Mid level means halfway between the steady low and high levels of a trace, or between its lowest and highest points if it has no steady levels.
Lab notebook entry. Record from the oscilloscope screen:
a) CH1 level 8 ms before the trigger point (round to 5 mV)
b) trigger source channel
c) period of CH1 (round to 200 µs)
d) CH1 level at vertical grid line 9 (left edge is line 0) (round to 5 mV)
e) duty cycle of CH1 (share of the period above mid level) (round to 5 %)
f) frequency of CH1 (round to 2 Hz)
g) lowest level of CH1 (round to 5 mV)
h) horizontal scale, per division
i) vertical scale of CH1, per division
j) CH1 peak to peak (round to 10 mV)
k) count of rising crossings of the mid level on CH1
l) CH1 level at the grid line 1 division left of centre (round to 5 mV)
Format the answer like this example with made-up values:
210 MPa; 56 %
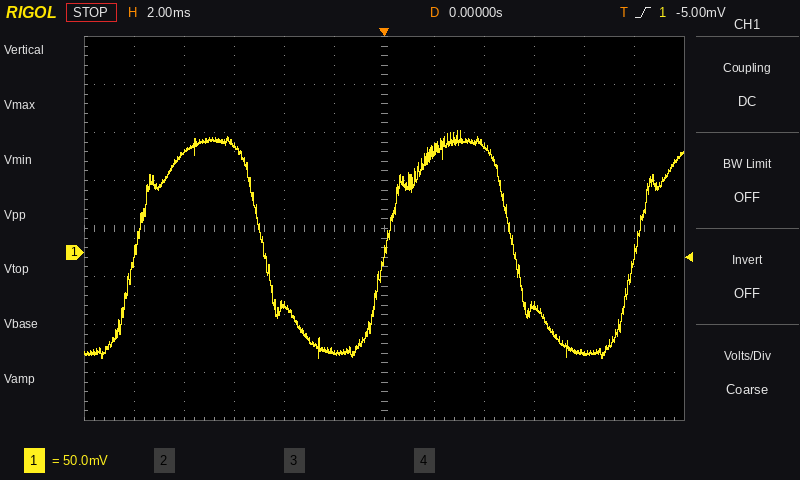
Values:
105 mV; CH1; 10.0 ms; -55 mV; 50 %; 100 Hz; -110 mV; 2 ms; 50 mV; 240 mV; 3; -105 mV
